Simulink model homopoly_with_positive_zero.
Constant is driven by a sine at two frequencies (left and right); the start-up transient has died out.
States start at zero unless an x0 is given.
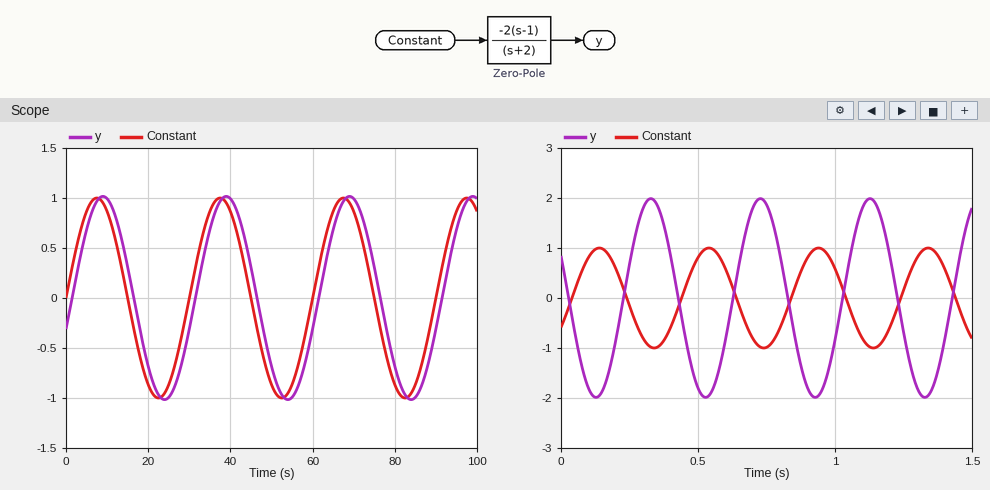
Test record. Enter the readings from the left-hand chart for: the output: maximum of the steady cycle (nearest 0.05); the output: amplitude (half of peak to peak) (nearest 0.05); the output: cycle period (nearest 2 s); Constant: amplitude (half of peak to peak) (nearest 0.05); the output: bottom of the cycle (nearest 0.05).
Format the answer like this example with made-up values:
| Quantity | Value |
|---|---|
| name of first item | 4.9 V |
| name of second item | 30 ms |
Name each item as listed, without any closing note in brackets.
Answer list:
| Quantity | Value |
|---|---|
| the output: maximum of the steady cycle | 1.00 |
| the output: amplitude (half of peak to peak) | 1.00 |
| the output: cycle period | 30 s |
| Constant: amplitude (half of peak to peak) | 1.00 |
| the output: bottom of the cycle | -1.00 |
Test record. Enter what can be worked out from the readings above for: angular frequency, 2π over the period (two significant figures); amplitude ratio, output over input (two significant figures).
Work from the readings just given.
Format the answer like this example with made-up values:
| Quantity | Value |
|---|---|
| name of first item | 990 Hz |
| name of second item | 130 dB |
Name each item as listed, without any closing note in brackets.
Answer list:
| Quantity | Value |
|---|---|
| angular frequency, 2π over the period | 0.21 rad/s |
| amplitude ratio, output over input | 1.0 |
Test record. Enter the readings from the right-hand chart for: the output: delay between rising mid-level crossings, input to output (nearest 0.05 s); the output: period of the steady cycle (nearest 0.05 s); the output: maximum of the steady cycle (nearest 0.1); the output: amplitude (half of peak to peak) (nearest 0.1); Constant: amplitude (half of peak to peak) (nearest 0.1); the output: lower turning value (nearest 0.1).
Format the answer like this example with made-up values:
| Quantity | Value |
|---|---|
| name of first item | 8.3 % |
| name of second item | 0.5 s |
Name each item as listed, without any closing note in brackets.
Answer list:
| Quantity | Value |
|---|---|
| the output: delay between rising mid-level crossings, input to output | 0.20 s |
| the output: period of the steady cycle | 0.40 s |
| the output: maximum of the steady cycle | 2.0 |
| the output: amplitude (half of peak to peak) | 2.0 |
| Constant: amplitude (half of peak to peak) | 1.0 |
| the output: lower turning value | -2.0 |
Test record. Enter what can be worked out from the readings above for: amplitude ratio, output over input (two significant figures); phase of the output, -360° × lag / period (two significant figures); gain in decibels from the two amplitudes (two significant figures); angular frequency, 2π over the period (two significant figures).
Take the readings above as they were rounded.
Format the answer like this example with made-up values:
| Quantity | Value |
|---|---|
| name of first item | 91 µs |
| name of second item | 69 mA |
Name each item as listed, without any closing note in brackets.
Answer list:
| Quantity | Value |
|---|---|
| amplitude ratio, output over input | 2.0 |
| phase of the output, -360° × lag / period | -180° |
| gain in decibels from the two amplitudes | 6.0 dB |
| angular frequency, 2π over the period | 16 rad/s |
